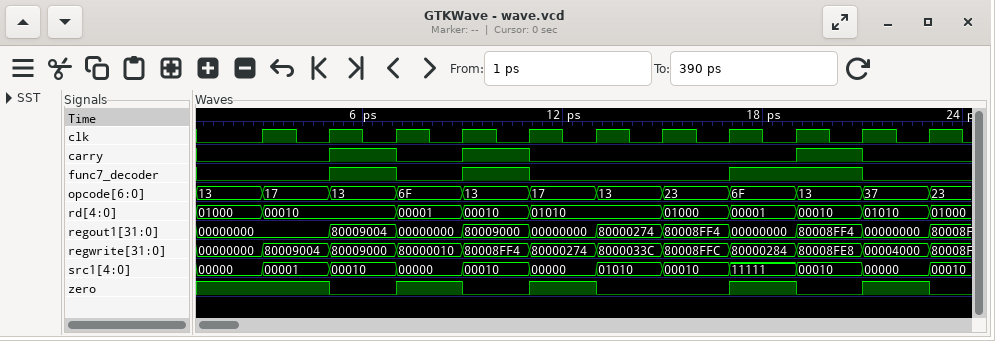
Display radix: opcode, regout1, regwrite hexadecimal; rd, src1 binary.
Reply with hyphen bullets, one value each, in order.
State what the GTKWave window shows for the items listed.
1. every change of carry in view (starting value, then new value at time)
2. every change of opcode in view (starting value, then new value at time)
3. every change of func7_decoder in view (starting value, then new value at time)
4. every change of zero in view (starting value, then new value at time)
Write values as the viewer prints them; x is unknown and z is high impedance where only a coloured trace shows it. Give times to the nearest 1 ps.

- 0, 1 at 5 ps, 0 at 7 ps, 1 at 9 ps, 0 at 11 ps, 1 at 19 ps, 0 at 21 ps
- 13, 17 at 3 ps, 13 at 5 ps, 6F at 7 ps, 13 at 9 ps, 17 at 11 ps, 13 at 13 ps, 23 at 15 ps, 6F at 17 ps, 13 at 19 ps, 37 at 21 ps, 23 at 23 ps
- 0, 1 at 5 ps, 0 at 7 ps, 1 at 9 ps, 0 at 11 ps, 1 at 17 ps, 0 at 21 ps
- 1, 0 at 5 ps, 1 at 7 ps, 0 at 9 ps, 1 at 11 ps, 0 at 13 ps, 1 at 17 ps, 0 at 19 ps, 1 at 21 ps, 0 at 23 ps
